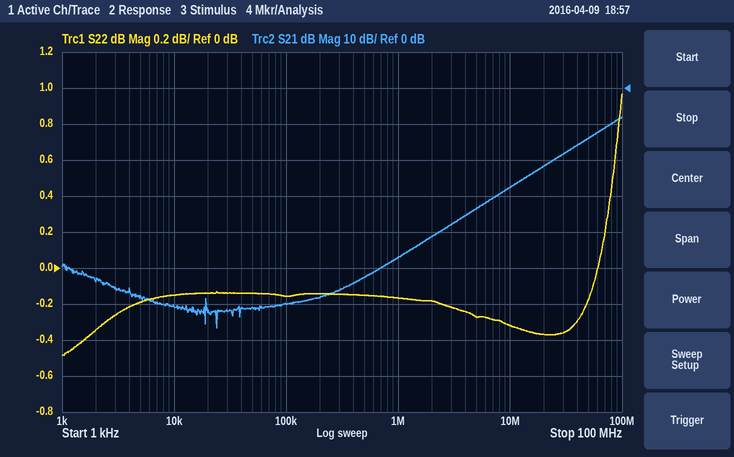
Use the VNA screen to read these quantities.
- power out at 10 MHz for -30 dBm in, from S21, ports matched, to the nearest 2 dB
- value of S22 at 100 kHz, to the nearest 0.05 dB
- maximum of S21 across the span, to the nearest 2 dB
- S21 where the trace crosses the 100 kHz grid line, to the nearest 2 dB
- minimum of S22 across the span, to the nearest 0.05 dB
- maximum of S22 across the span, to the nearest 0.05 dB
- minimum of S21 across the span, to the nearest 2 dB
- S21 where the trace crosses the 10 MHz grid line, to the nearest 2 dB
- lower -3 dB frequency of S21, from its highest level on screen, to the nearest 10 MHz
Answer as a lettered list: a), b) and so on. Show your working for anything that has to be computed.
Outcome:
a) -30 dBm + (-28 dB) = -58 dBm
b) -0.15 dB
c) -8 dB
d) -60 dB
e) -0.50 dB
f) 0.95 dB
g) -66 dB
h) -28 dB
i) 70 MHz
